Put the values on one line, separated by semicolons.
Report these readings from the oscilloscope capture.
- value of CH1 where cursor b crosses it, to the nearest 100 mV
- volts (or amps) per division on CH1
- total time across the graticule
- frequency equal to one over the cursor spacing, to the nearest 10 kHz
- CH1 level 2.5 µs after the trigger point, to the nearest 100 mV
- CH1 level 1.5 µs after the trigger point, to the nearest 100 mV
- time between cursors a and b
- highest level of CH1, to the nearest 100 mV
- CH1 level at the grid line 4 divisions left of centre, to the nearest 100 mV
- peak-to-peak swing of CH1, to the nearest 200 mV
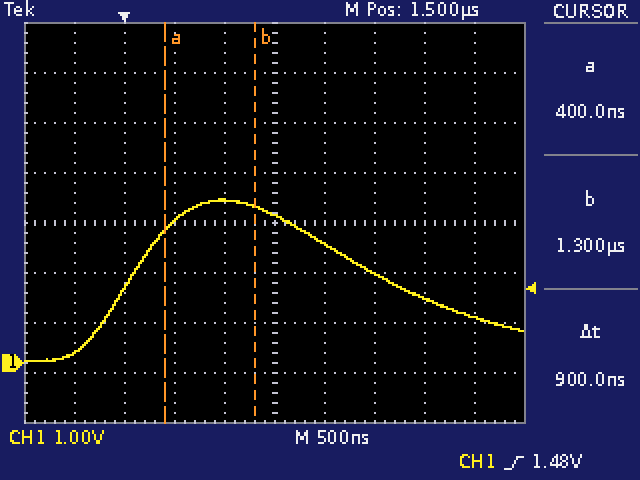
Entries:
3.1 V; 1 V; 5 µs; 1.11 MHz; 1.8 V; 3.0 V; 900 ns; 3.3 V; 200 mV; 3.2 V
